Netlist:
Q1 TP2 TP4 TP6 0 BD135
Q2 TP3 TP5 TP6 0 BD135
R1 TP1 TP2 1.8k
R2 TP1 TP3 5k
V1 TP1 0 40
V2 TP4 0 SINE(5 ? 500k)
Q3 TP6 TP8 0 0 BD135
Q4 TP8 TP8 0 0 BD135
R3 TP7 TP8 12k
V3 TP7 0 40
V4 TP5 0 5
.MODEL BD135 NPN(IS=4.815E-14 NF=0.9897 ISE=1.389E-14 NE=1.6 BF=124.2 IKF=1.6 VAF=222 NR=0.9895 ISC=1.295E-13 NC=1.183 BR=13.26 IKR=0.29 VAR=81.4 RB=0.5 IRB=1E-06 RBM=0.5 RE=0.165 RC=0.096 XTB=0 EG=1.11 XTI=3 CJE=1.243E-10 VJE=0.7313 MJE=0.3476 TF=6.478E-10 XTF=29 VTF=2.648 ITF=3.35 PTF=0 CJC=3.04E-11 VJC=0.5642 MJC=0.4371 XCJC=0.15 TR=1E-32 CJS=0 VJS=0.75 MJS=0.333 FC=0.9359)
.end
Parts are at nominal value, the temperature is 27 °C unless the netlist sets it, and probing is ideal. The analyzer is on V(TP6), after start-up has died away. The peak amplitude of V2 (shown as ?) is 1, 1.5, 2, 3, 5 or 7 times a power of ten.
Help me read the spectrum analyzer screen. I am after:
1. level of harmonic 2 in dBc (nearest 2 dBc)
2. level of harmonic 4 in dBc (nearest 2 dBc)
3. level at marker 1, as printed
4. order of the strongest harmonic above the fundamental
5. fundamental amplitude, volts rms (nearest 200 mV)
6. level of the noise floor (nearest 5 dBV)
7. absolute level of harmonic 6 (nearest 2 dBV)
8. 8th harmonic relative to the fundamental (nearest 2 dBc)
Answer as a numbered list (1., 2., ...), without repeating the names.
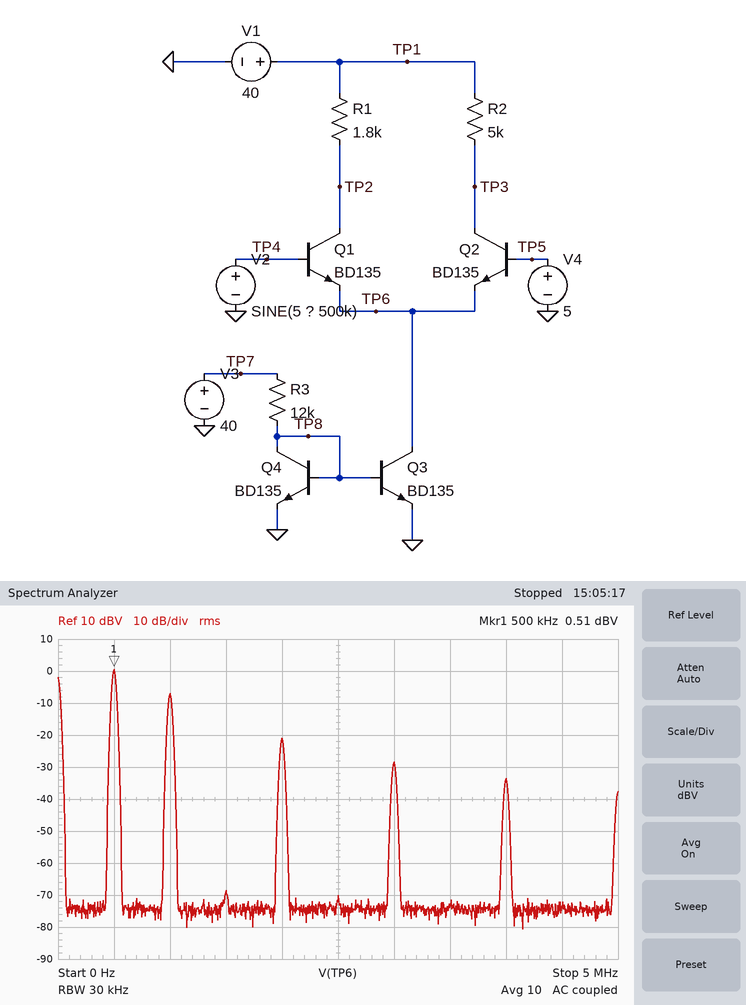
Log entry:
1. -8 dBc
2. -22 dBc
3. 0.51 dBV
4. 2
5. 1.0 V
6. -75 dBV
7. -28 dBV
8. -34 dBc
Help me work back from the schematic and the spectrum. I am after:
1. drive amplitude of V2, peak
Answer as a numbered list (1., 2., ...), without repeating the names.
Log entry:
1. 3 V
